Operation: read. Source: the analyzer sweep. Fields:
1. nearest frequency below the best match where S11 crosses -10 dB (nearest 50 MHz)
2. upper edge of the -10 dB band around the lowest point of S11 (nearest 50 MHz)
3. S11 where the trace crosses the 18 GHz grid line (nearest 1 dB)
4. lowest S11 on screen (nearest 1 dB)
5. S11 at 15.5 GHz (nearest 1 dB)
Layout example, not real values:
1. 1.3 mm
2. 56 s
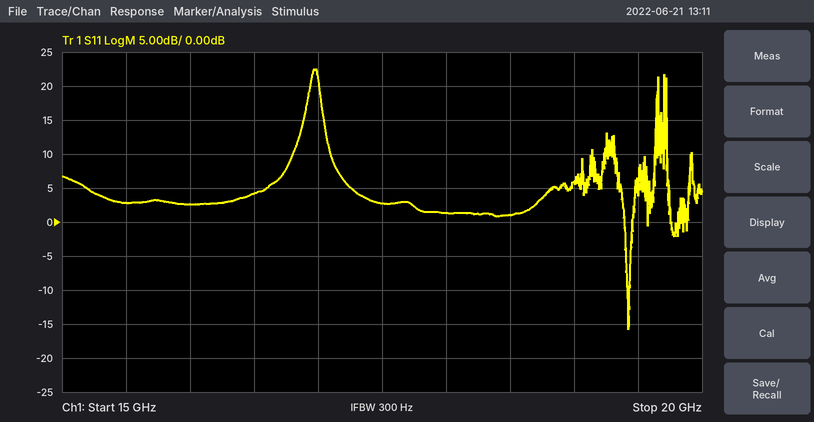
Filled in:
1. 19.40 GHz
2. 19.45 GHz
3. 1 dB
4. -16 dB
5. 3 dB
